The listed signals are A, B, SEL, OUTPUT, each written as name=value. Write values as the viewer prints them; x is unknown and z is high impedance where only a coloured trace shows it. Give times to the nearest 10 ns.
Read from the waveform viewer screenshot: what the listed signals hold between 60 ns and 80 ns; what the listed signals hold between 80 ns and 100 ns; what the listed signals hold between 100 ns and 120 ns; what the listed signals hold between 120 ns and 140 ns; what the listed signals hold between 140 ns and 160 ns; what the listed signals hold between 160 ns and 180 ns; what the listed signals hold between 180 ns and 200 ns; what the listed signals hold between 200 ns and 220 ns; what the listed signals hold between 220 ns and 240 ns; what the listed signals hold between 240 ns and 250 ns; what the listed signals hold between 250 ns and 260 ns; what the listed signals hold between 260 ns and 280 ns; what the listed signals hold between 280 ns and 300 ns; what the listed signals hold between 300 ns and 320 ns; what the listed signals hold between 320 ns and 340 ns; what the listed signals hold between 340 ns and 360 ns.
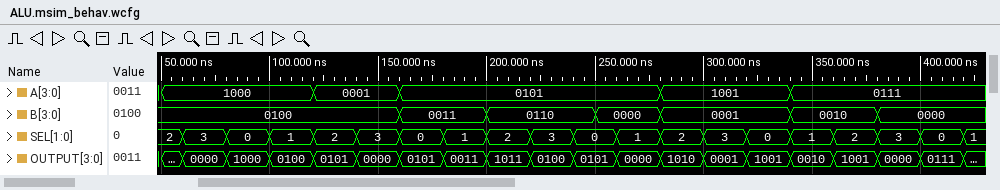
A=1000, B=0100, SEL=3, OUTPUT=0000
A=1000, B=0100, SEL=0, OUTPUT=1000
A=1000, B=0100, SEL=1, OUTPUT=0100
A=0001, B=0100, SEL=2, OUTPUT=0101
A=0001, B=0100, SEL=3, OUTPUT=0000
A=0101, B=0011, SEL=0, OUTPUT=0101
A=0101, B=0011, SEL=1, OUTPUT=0011
A=0101, B=0110, SEL=2, OUTPUT=1011
A=0101, B=0110, SEL=3, OUTPUT=0100
A=0101, B=0110, SEL=0, OUTPUT=0101
A=0101, B=0000, SEL=0, OUTPUT=0101
A=0101, B=0000, SEL=1, OUTPUT=0000
A=1001, B=0001, SEL=2, OUTPUT=1010
A=1001, B=0001, SEL=3, OUTPUT=0001
A=1001, B=0001, SEL=0, OUTPUT=1001
A=0111, B=0010, SEL=1, OUTPUT=0010
